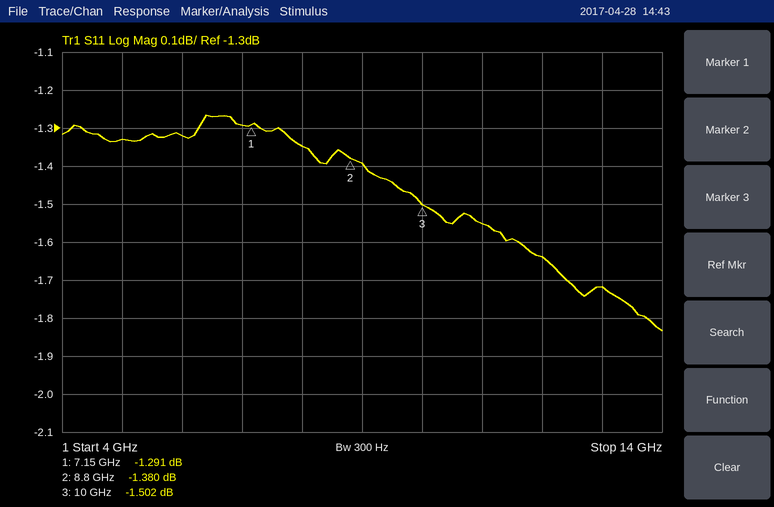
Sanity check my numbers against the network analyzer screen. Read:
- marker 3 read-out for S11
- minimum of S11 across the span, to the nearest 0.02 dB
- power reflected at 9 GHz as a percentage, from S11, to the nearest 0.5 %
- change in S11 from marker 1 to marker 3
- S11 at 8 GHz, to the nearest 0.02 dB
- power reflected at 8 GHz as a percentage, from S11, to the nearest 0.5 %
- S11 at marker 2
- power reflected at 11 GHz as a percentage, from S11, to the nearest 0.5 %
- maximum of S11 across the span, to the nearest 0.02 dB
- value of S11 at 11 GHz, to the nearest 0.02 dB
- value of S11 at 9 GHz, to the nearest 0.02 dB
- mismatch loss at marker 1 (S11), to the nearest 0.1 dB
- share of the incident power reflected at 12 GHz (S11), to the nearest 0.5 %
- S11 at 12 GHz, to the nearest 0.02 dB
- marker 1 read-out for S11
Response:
-1.502 dB
-1.84 dB
72.5 %
-0.211 dB
-1.34 dB
73.5 %
-1.380 dB
70.0 %
-1.26 dB
-1.56 dB
-1.40 dB
5.9 dB
68.5 %
-1.64 dB
-1.291 dB
